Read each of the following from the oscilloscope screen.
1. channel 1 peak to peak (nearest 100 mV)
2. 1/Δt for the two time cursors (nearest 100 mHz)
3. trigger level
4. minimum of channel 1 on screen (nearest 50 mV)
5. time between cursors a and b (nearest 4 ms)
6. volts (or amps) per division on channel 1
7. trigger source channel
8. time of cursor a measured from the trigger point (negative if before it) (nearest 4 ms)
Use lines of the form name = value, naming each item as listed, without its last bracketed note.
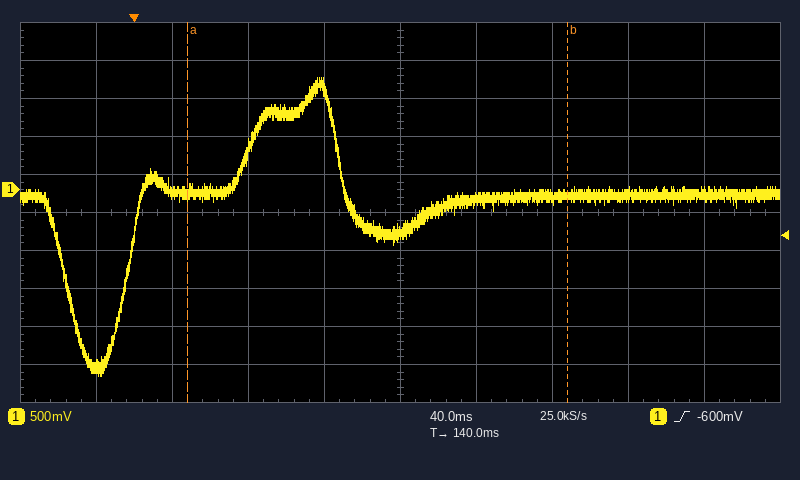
channel 1 peak to peak = 3.90 V
1/Δt for the two time cursors = 5.0 Hz
trigger level = -600 mV
minimum of channel 1 on screen = -2.45 V
time between cursors a and b = 200 ms
volts (or amps) per division on channel 1 = 500 mV
trigger source channel = channel 1
time of cursor a measured from the trigger point (negative if before it) = +28 ms
